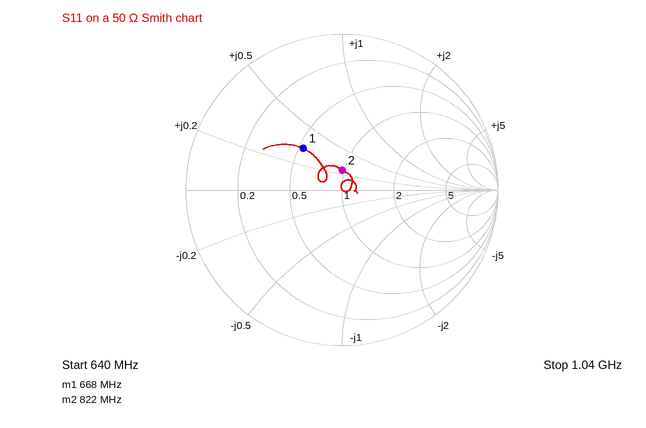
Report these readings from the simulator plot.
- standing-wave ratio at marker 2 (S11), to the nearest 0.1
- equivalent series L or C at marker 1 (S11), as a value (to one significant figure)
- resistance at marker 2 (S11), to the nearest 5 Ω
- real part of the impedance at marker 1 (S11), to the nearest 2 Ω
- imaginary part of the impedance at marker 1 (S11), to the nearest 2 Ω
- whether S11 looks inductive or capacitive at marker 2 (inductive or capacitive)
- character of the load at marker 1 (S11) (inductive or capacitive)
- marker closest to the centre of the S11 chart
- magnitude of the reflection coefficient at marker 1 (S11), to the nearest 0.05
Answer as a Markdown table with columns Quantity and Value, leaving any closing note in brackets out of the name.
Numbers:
| Quantity | Value |
|---|---|
| standing-wave ratio at marker 2 (S11), to the nearest 0.1 | 1.3 |
| equivalent series L or C at marker 1 (S11), as a value | 4 nH |
| resistance at marker 2 (S11), to the nearest 5 Ω | 50 Ω |
| real part of the impedance at marker 1 (S11), to the nearest 2 Ω | 26 Ω |
| imaginary part of the impedance at marker 1 (S11), to the nearest 2 Ω | +16 Ω |
| whether S11 looks inductive or capacitive at marker 2 | inductive |
| character of the load at marker 1 (S11) | inductive |
| marker closest to the centre of the S11 chart | marker 2 |
| magnitude of the reflection coefficient at marker 1 (S11), to the nearest 0.05 | 0.35 |
